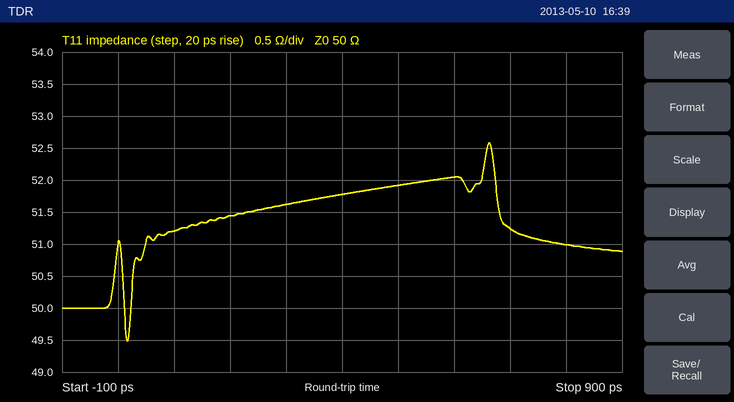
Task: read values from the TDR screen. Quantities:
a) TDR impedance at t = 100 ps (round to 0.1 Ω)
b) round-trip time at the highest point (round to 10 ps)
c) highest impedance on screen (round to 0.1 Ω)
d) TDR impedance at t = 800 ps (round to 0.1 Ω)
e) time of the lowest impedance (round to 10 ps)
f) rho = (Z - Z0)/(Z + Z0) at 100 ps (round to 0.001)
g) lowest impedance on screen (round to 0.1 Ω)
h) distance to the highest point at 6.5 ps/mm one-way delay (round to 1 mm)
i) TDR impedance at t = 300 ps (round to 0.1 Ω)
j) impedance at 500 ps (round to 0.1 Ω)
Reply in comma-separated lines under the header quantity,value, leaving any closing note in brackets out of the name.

quantity,value
TDR impedance at t = 100 ps,51.2 Ω
round-trip time at the highest point,660 ps
highest impedance on screen,52.6 Ω
TDR impedance at t = 800 ps,51.0 Ω
time of the lowest impedance,20 ps
rho = (Z - Z0)/(Z + Z0) at 100 ps,+0.012
lowest impedance on screen,49.5 Ω
distance to the highest point at 6.5 ps/mm one-way delay,51 mm
TDR impedance at t = 300 ps,51.6 Ω
impedance at 500 ps,51.9 Ω
